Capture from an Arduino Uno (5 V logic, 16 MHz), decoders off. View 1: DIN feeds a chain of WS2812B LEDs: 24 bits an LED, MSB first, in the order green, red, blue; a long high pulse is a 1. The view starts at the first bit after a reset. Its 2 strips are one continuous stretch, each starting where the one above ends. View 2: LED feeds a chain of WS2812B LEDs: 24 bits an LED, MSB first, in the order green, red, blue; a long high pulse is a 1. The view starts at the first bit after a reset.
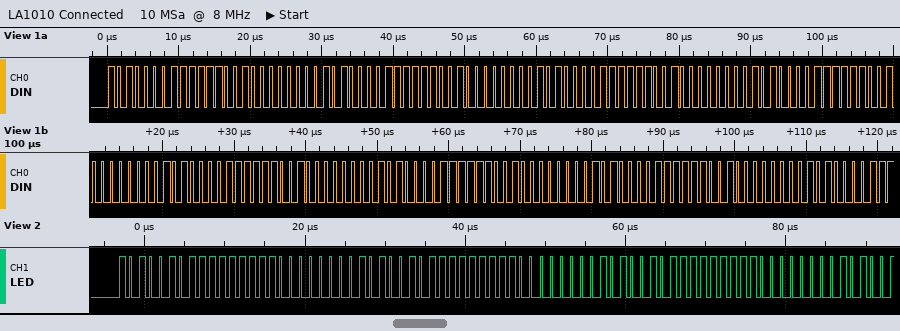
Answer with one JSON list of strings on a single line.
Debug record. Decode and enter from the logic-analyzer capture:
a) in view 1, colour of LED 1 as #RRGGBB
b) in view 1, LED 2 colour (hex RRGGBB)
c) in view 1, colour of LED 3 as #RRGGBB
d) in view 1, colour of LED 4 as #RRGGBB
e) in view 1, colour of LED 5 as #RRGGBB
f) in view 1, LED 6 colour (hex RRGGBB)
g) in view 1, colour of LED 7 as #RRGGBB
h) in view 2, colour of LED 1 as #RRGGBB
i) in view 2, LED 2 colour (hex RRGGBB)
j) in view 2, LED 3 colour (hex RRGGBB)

["#F9A100", "#F9A100", "#F9A100", "#F9A100", "#F9A100", "#F9A100", "#F9A100", "#FFA500", "#FFA500", "#FFA500"]
